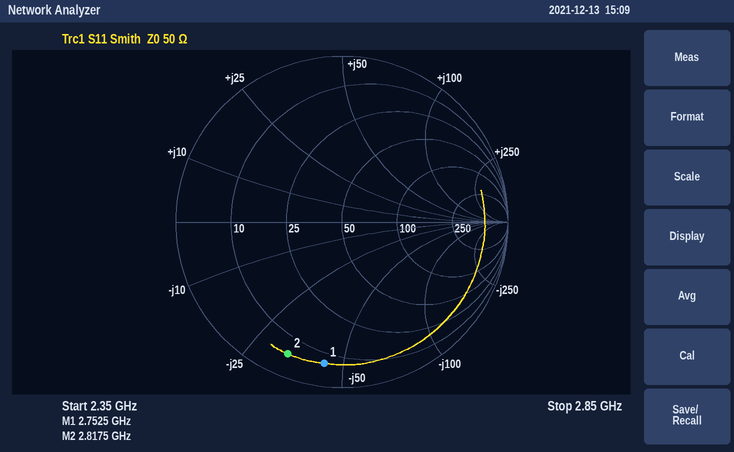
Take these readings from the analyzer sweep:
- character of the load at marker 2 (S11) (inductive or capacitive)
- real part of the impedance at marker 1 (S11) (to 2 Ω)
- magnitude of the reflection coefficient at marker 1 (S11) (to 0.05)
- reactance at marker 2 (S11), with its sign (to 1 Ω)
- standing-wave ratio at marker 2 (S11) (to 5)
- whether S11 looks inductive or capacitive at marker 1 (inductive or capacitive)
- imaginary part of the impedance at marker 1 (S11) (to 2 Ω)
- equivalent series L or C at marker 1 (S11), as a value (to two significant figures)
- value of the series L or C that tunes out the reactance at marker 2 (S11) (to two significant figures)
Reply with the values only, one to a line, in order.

capacitive
6 Ω
0.85
-33 Ω
15
capacitive
-44 Ω
1.3 pF
1.9 nH
